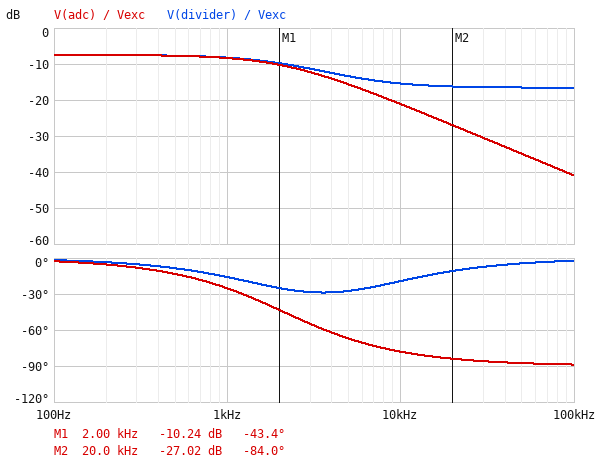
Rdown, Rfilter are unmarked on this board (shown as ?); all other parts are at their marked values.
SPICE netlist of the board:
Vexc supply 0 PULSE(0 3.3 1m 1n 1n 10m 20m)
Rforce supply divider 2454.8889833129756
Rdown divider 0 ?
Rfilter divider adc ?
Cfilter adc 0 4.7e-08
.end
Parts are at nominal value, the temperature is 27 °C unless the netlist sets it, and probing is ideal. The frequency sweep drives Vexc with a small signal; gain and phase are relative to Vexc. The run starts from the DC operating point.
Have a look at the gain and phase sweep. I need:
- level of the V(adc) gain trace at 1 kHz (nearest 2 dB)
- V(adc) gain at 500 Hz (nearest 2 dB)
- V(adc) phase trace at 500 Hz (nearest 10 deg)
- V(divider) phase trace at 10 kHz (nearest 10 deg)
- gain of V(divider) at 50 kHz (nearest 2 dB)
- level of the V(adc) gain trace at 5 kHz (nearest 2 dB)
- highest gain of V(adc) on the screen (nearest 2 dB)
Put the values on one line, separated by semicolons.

-8 dB; -8 dB; -10 deg; -20 deg; -16 dB; -16 dB; -8 dB
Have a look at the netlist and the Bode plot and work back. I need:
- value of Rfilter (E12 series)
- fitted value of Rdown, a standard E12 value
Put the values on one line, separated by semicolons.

560 Ω; 1.8 kΩ
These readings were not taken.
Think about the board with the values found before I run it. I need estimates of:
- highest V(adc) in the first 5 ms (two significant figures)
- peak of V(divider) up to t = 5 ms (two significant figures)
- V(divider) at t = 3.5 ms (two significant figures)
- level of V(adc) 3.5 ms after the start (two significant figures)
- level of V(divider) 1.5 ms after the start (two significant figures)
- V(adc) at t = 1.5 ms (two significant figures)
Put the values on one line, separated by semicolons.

1.4 V; 1.4 V; 1.4 V; 1.4 V; 1.4 V; 1.4 V
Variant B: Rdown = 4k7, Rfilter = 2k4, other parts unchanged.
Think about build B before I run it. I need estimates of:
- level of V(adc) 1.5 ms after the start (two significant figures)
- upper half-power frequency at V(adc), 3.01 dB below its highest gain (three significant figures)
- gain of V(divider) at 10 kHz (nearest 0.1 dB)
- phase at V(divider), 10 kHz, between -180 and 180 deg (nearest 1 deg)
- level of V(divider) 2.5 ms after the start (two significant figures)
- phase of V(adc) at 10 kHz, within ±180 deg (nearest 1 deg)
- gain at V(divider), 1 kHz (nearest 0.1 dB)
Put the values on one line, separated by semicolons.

2.0 V; 844 Hz; -8.1 dB; -3 deg; 2.2 V; -85 deg; -5.7 dB
